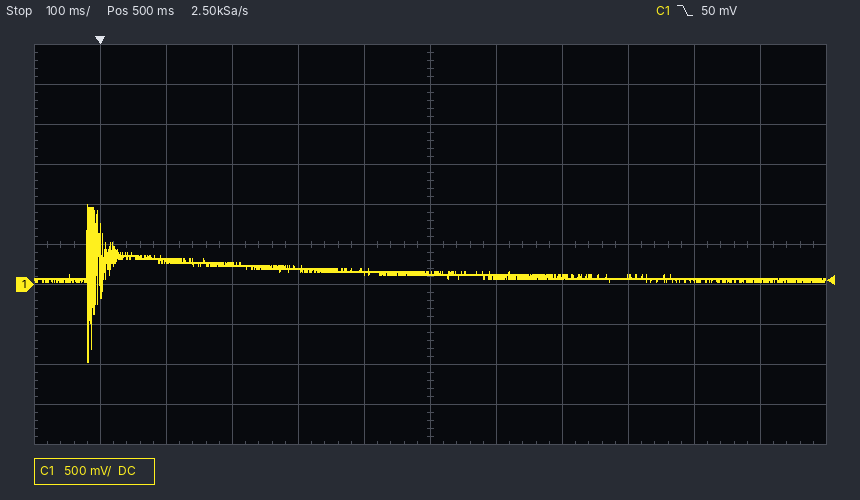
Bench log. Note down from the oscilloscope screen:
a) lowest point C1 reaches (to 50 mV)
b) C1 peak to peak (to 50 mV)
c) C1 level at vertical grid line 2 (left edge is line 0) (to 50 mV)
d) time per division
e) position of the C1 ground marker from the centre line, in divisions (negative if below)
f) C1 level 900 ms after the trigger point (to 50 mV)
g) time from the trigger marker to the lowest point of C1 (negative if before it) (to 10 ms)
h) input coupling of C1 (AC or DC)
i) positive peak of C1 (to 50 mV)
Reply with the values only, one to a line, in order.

-950 mV
1.95 V
300 mV
100 ms
-1.0 div
50 mV
-20 ms
DC
1.00 V
